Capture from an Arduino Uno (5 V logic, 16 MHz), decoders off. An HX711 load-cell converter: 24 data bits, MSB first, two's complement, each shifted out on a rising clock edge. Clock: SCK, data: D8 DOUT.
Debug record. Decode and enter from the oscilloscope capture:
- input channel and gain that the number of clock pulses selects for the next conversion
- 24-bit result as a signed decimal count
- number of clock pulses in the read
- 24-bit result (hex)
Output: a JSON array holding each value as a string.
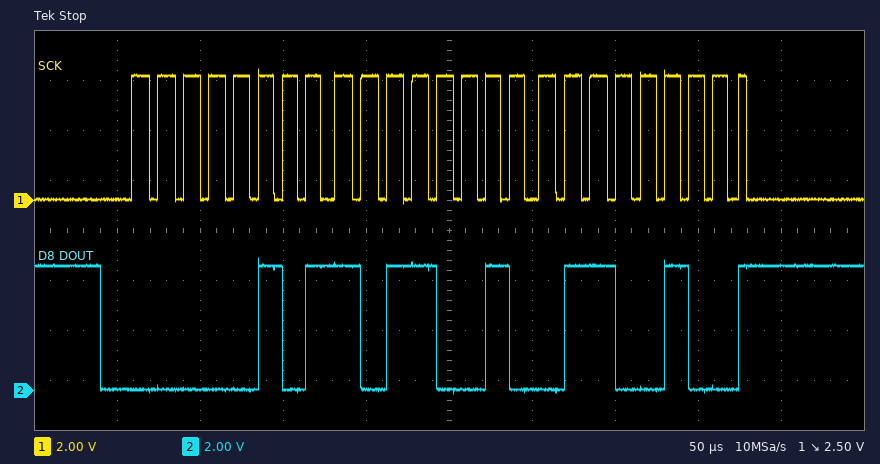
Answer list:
["channel A, gain 128", "373348", "25", "0x05B264"]
